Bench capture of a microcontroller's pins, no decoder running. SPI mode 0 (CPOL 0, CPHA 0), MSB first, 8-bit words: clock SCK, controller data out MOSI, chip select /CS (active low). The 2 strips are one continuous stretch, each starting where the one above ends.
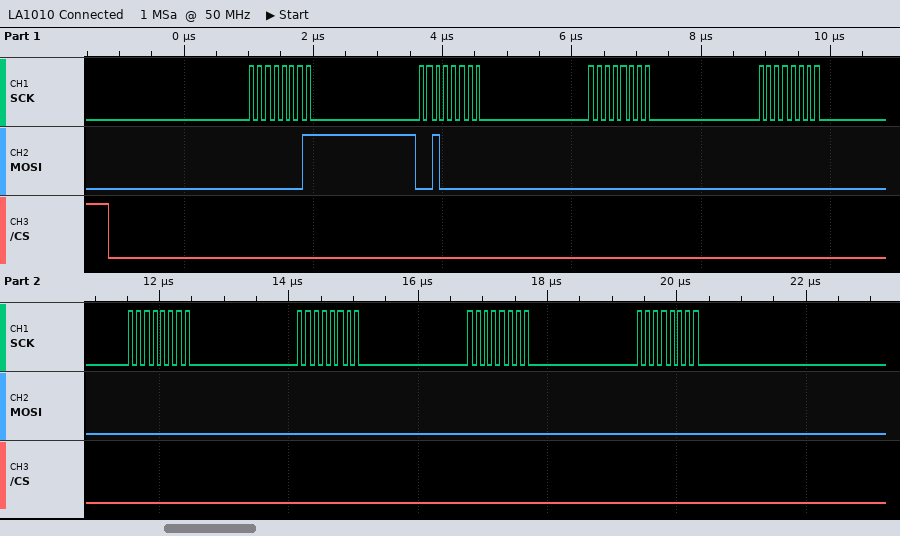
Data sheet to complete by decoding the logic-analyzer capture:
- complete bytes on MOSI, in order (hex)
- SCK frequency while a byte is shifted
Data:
01 20 00 00 00 00 00 00
8 MHz
